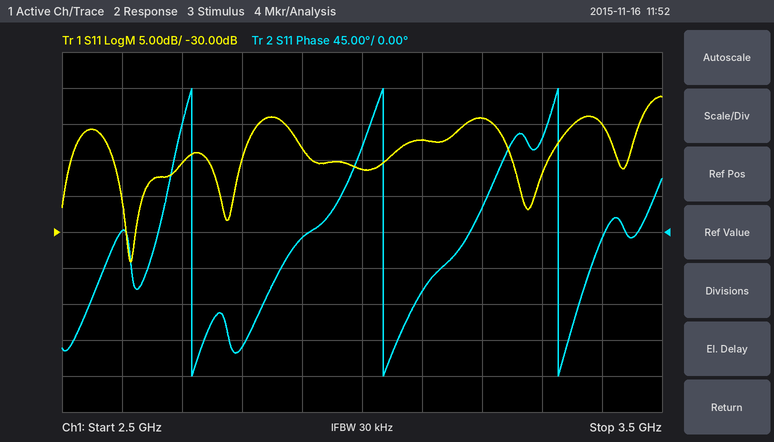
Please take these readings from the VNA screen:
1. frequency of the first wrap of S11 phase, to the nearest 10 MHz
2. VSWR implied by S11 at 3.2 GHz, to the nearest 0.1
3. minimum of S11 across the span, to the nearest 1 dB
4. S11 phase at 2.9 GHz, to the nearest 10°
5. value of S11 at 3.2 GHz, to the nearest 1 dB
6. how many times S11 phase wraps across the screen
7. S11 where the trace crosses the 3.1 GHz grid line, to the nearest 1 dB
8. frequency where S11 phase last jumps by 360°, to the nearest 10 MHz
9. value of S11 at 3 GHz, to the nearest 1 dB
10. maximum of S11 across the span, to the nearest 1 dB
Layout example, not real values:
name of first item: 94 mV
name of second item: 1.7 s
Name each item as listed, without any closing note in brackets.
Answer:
frequency of the first wrap of S11 phase, to the nearest 10 MHz: 2.72 GHz
VSWR implied by S11 at 3.2 GHz, to the nearest 0.1: 1.5
minimum of S11 across the span, to the nearest 1 dB: -34 dB
S11 phase at 2.9 GHz, to the nearest 10°: -10°
value of S11 at 3.2 GHz, to the nearest 1 dB: -14 dB
how many times S11 phase wraps across the screen: 3
S11 where the trace crosses the 3.1 GHz grid line, to the nearest 1 dB: -17 dB
frequency where S11 phase last jumps by 360°, to the nearest 10 MHz: 3.33 GHz
value of S11 at 3 GHz, to the nearest 1 dB: -21 dB
maximum of S11 across the span, to the nearest 1 dB: -11 dB
